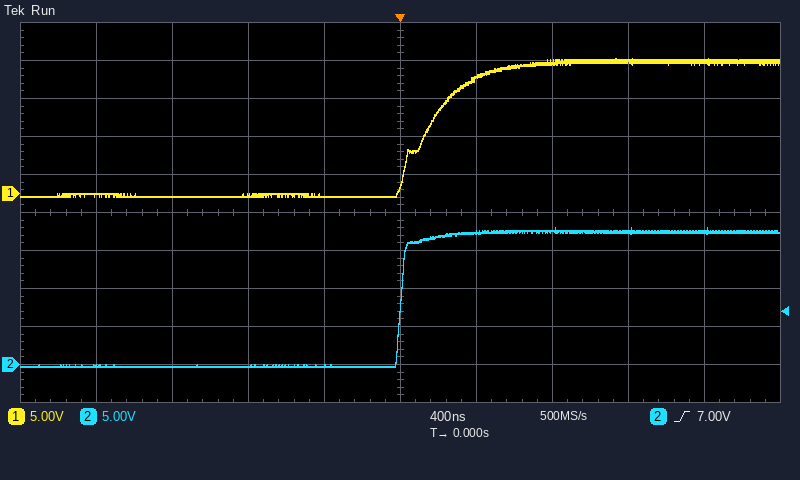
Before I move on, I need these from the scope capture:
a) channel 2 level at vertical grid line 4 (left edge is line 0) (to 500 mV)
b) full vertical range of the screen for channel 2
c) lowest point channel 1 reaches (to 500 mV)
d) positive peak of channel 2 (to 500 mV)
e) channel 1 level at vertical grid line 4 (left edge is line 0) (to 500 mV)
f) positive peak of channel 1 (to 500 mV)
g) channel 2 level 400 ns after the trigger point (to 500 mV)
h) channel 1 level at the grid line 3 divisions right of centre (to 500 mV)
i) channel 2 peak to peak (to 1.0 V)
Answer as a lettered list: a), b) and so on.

a) 0.0 V
b) 50 V
c) -500 mV
d) 18.0 V
e) -500 mV
f) 18.0 V
g) 17.5 V
h) 17.5 V
i) 18.0 V
